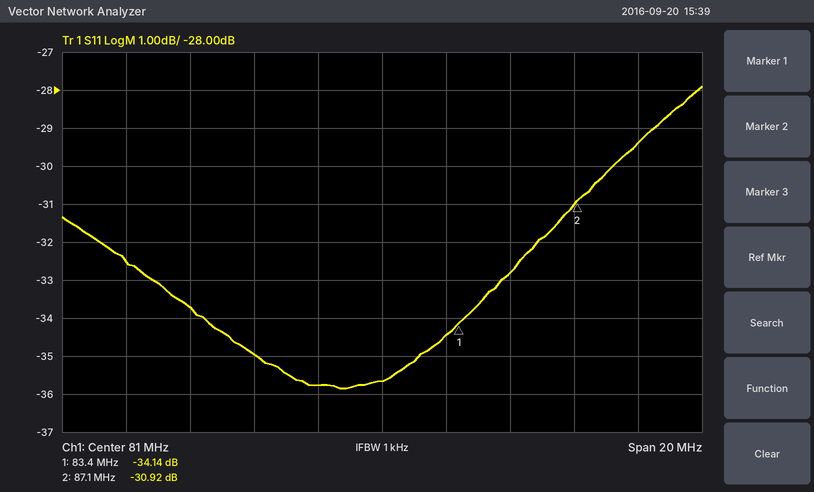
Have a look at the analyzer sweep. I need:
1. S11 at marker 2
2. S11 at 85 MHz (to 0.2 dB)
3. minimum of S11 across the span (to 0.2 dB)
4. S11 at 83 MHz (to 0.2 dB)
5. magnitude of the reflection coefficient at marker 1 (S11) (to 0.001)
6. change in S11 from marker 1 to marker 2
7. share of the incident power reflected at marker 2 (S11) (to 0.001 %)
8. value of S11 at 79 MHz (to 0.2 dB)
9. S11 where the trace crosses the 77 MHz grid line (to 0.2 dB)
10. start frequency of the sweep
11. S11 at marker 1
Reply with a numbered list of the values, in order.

1. -30.92 dB
2. -32.8 dB
3. -35.8 dB
4. -34.4 dB
5. 0.020
6. 3.22 dB
7. 0.081 %
8. -35.8 dB
9. -35.0 dB
10. 71 MHz
11. -34.14 dB
